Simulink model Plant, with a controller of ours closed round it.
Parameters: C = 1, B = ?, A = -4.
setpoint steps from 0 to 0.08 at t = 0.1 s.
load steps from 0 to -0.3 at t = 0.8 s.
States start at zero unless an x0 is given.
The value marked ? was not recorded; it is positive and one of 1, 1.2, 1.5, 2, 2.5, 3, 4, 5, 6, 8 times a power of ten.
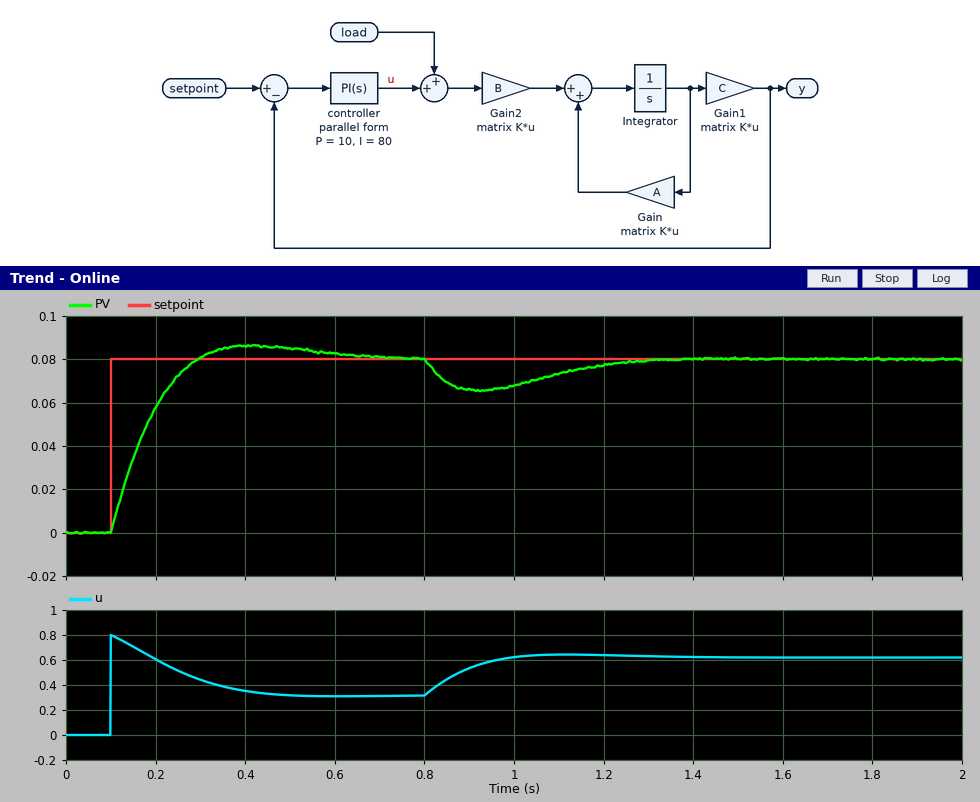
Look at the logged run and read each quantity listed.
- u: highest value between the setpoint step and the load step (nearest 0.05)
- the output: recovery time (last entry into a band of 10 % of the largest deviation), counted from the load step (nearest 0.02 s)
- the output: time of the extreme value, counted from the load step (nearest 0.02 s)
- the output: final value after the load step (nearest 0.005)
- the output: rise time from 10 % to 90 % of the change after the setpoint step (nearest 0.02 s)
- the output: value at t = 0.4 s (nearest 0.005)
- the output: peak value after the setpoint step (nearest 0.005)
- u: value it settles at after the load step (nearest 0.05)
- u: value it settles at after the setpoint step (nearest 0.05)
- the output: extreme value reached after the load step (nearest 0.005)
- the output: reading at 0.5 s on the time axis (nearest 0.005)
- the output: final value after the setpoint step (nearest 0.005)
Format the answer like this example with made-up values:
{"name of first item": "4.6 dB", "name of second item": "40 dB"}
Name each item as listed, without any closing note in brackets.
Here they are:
{"u: highest value between the setpoint step and the load step": "0.80", "the output: recovery time (last entry into a band of 10 % of the largest deviation), counted from the load step": "0.44 s", "the output: time of the extreme value, counted from the load step": "0.12 s", "the output: final value after the load step": "0.080", "the output: rise time from 10 % to 90 % of the change after the setpoint step": "0.14 s", "the output: value at t = 0.4 s": "0.085", "the output: peak value after the setpoint step": "0.085", "u: value it settles at after the load step": "0.60", "u: value it settles at after the setpoint step": "0.30", "the output: extreme value reached after the load step": "0.065", "the output: reading at 0.5 s on the time axis": "0.085", "the output: final value after the setpoint step": "0.080"}
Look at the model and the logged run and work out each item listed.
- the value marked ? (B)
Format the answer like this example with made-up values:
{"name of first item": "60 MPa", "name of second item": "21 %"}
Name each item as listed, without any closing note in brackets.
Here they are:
{"the value marked ?": "1"}
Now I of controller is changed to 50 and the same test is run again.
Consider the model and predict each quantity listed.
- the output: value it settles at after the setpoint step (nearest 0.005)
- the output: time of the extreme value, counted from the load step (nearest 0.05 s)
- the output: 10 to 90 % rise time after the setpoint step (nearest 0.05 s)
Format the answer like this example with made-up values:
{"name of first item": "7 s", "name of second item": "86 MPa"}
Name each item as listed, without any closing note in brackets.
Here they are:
{"the output: value it settles at after the setpoint step": "0.080", "the output: time of the extreme value, counted from the load step": "0.15 s", "the output: 10 to 90 % rise time after the setpoint step": "0.20 s"}
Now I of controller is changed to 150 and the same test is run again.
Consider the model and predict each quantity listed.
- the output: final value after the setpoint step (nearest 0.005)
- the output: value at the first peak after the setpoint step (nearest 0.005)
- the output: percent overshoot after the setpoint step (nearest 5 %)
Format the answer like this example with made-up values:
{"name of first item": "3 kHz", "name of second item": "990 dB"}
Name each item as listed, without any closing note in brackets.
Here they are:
{"the output: final value after the setpoint step": "0.080", "the output: value at the first peak after the setpoint step": "0.095", "the output: percent overshoot after the setpoint step": "20 %"}
